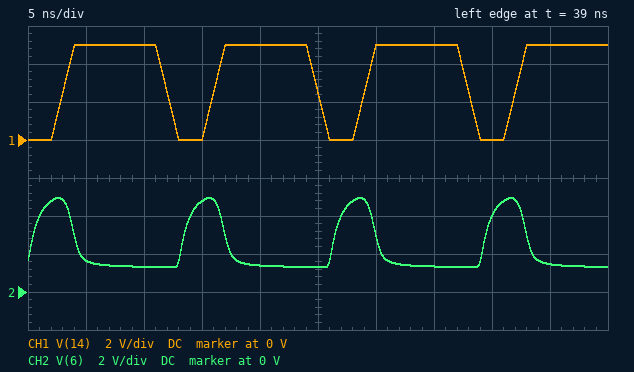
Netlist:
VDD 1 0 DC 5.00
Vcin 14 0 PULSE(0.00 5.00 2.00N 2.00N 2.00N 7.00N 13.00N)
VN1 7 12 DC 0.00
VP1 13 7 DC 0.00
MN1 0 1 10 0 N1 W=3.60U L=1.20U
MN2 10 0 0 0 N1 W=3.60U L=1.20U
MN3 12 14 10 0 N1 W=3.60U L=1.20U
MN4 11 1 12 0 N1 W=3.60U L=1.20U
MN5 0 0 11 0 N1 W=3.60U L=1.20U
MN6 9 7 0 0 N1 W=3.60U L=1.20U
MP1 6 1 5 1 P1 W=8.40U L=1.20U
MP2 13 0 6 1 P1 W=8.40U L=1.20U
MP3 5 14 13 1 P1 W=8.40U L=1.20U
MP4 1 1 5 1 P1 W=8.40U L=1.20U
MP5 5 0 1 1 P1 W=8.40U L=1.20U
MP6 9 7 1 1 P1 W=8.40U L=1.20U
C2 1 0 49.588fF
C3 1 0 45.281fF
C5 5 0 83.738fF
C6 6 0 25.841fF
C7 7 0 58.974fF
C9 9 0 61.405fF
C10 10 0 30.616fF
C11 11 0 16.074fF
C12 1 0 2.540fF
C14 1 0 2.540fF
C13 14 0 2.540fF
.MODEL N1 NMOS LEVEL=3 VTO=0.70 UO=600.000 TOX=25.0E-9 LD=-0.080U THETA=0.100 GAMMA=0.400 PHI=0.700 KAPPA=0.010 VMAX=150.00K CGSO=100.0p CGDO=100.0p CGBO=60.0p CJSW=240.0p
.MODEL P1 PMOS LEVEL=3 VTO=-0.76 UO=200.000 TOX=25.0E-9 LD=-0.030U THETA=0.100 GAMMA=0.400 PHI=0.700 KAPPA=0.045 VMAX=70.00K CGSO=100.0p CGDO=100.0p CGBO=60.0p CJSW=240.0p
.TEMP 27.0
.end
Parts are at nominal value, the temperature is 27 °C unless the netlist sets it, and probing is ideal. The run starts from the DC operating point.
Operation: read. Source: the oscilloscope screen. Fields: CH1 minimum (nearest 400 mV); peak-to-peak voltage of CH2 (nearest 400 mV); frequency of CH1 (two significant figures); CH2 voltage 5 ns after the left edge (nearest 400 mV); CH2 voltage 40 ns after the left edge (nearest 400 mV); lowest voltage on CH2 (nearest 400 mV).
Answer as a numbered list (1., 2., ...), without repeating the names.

1. 0 V
2. 3.6 V
3. 77 MHz
4. 1.6 V
5. 4.0 V
6. 1.2 V
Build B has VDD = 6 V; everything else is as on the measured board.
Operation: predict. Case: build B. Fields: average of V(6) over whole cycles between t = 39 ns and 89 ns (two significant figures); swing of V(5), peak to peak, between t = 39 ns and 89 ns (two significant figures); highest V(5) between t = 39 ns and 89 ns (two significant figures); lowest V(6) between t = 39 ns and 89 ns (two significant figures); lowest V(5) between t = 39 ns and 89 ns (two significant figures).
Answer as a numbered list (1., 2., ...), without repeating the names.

1. 2.8 V
2. 1.1 V
3. 6.0 V
4. 1.4 V
5. 4.9 V
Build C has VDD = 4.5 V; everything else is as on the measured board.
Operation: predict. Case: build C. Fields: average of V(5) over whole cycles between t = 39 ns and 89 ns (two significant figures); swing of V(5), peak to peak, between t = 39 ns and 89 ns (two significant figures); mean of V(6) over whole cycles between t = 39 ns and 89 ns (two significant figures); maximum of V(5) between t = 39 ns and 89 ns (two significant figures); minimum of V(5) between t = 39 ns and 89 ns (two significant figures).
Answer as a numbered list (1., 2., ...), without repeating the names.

1. 4.4 V
2. 860 mV
3. 2.0 V
4. 4.5 V
5. 3.7 V
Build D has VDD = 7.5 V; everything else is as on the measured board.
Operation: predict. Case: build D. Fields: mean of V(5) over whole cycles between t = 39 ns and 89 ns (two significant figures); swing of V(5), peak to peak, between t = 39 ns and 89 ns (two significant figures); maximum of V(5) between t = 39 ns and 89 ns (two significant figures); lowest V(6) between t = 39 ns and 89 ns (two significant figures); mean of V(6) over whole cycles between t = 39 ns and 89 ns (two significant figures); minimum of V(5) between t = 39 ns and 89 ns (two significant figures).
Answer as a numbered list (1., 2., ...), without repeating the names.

1. 7.2 V
2. 1.2 V
3. 7.5 V
4. 1.5 V
5. 3.7 V
6. 6.3 V
